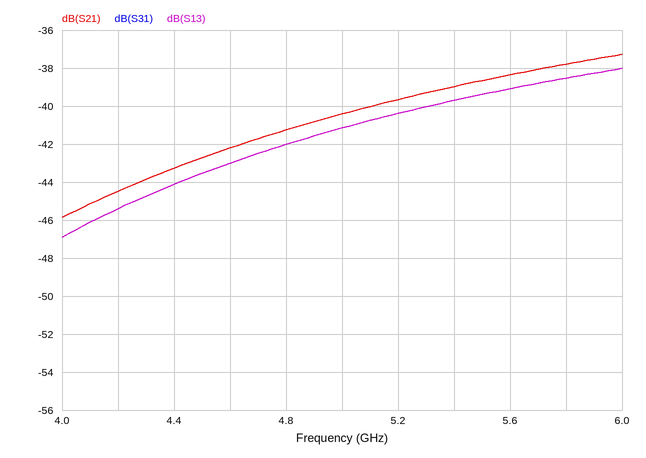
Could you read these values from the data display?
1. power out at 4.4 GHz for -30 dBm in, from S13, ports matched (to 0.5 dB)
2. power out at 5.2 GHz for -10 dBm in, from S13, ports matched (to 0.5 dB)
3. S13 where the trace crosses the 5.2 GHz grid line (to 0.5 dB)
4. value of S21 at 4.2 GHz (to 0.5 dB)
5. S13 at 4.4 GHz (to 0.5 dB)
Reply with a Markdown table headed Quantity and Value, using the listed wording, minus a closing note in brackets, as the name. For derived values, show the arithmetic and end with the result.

| Quantity | Value |
|---|---|
| power out at 4.4 GHz for -30 dBm in, from S13, ports matched | -30 dBm + (-44.0 dB) = -74.0 dBm |
| power out at 5.2 GHz for -10 dBm in, from S13, ports matched | -10 dBm + (-40.5 dB) = -50.5 dBm |
| S13 where the trace crosses the 5.2 GHz grid line | -40.5 dB |
| value of S21 at 4.2 GHz | -44.5 dB |
| S13 at 4.4 GHz | -44.0 dB |
